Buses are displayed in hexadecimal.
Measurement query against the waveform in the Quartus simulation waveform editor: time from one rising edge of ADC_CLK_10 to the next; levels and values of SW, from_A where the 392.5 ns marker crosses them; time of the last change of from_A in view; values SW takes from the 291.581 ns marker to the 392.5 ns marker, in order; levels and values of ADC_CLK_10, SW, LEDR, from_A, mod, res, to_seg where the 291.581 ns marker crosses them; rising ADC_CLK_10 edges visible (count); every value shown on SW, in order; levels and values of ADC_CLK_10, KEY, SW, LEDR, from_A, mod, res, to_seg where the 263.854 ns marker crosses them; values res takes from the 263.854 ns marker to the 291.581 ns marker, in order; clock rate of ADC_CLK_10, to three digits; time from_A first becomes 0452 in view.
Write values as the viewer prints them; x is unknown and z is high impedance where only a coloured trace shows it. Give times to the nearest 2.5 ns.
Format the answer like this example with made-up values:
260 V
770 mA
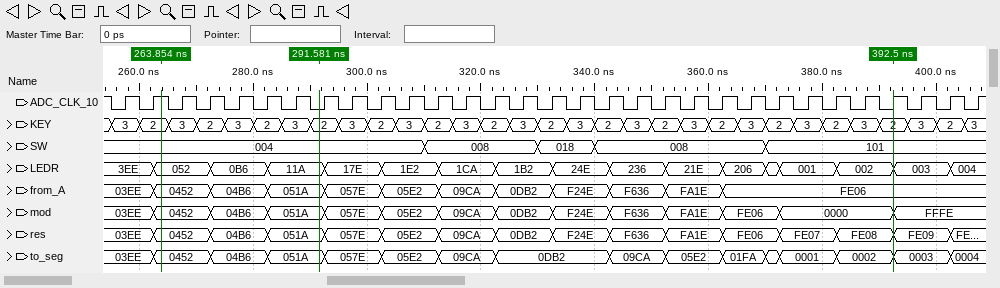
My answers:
5 ns
SW=101, from_A=FE06
362.5 ns
004, 008, 018, 008, 101
ADC_CLK_10=0, SW=004, LEDR=11A, from_A=051A, mod=051A, res=051A, to_seg=051A
31
004, 008, 018, 008, 101
ADC_CLK_10=1, KEY=2, SW=004, LEDR=052, from_A=0452, mod=0452, res=0452, to_seg=0452
0452, 04B6, 051A
200 MHz
262.5 ns
